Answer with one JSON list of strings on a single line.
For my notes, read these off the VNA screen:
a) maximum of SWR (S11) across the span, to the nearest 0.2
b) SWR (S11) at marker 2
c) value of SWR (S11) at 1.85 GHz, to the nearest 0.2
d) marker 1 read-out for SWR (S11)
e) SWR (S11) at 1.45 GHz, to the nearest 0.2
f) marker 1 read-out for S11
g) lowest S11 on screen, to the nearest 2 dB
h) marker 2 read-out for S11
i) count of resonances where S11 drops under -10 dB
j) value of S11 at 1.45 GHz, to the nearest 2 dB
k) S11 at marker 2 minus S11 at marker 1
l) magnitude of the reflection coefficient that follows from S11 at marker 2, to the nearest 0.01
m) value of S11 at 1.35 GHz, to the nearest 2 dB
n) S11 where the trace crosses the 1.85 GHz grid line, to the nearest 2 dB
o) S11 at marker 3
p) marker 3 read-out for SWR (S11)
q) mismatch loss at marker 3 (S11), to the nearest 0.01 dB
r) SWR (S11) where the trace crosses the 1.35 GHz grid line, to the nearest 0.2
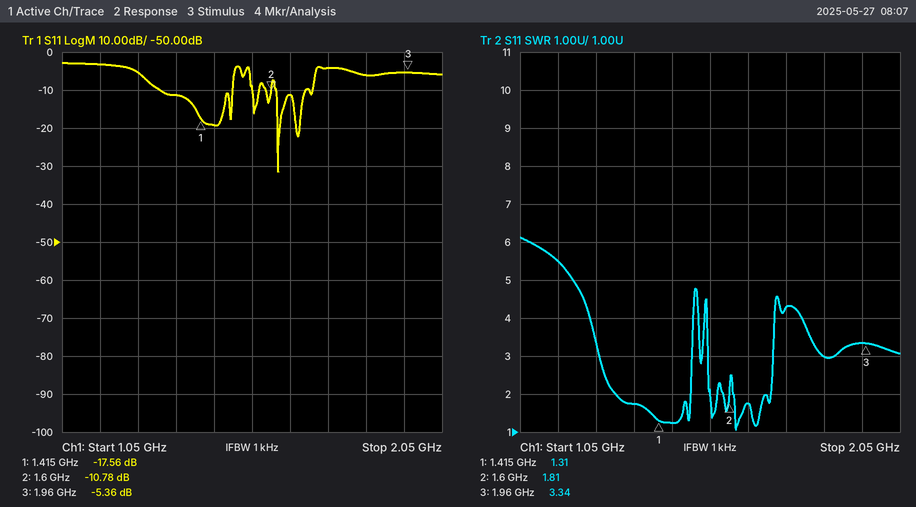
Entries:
["6.2", "1.81", "3.0", "1.31", "1.2", "-17.56 dB", "-32 dB", "-10.78 dB", "6", "-20 dB", "6.78 dB", "0.29", "-12 dB", "-6 dB", "-5.36 dB", "3.34", "1.49 dB", "1.8"]
